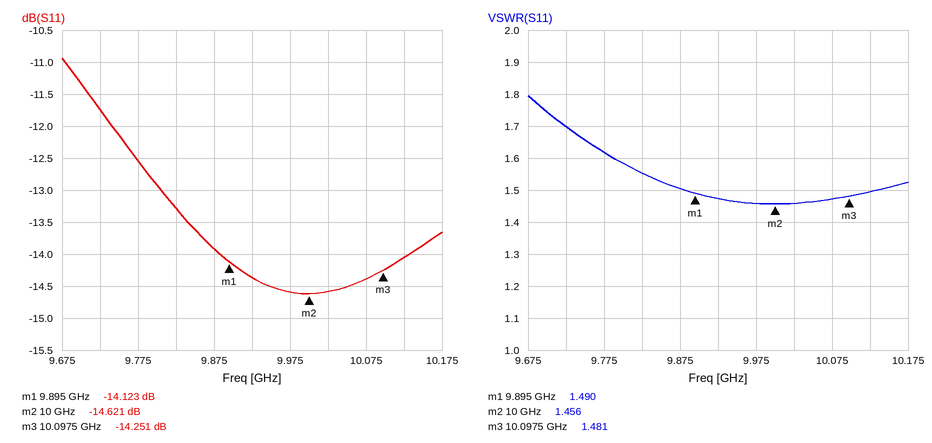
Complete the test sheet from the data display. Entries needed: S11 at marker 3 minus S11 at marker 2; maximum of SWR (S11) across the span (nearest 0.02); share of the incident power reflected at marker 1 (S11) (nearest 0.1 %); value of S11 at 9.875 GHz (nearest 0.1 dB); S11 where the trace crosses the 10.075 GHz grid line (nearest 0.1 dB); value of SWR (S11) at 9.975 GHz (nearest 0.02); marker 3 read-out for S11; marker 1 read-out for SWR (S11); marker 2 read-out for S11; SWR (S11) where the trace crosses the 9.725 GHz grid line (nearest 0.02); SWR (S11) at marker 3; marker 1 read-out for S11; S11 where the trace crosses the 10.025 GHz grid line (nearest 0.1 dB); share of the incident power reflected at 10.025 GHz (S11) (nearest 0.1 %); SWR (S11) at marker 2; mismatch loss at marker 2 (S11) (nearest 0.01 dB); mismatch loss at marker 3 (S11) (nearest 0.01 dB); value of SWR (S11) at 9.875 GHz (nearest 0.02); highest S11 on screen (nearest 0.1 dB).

0.370 dB
1.80
3.9 %
-13.9 dB
-14.4 dB
1.46
-14.251 dB
1.490
-14.621 dB
1.70
1.481
-14.123 dB
-14.6 dB
3.5 %
1.456
0.15 dB
0.17 dB
1.50
-10.9 dB
